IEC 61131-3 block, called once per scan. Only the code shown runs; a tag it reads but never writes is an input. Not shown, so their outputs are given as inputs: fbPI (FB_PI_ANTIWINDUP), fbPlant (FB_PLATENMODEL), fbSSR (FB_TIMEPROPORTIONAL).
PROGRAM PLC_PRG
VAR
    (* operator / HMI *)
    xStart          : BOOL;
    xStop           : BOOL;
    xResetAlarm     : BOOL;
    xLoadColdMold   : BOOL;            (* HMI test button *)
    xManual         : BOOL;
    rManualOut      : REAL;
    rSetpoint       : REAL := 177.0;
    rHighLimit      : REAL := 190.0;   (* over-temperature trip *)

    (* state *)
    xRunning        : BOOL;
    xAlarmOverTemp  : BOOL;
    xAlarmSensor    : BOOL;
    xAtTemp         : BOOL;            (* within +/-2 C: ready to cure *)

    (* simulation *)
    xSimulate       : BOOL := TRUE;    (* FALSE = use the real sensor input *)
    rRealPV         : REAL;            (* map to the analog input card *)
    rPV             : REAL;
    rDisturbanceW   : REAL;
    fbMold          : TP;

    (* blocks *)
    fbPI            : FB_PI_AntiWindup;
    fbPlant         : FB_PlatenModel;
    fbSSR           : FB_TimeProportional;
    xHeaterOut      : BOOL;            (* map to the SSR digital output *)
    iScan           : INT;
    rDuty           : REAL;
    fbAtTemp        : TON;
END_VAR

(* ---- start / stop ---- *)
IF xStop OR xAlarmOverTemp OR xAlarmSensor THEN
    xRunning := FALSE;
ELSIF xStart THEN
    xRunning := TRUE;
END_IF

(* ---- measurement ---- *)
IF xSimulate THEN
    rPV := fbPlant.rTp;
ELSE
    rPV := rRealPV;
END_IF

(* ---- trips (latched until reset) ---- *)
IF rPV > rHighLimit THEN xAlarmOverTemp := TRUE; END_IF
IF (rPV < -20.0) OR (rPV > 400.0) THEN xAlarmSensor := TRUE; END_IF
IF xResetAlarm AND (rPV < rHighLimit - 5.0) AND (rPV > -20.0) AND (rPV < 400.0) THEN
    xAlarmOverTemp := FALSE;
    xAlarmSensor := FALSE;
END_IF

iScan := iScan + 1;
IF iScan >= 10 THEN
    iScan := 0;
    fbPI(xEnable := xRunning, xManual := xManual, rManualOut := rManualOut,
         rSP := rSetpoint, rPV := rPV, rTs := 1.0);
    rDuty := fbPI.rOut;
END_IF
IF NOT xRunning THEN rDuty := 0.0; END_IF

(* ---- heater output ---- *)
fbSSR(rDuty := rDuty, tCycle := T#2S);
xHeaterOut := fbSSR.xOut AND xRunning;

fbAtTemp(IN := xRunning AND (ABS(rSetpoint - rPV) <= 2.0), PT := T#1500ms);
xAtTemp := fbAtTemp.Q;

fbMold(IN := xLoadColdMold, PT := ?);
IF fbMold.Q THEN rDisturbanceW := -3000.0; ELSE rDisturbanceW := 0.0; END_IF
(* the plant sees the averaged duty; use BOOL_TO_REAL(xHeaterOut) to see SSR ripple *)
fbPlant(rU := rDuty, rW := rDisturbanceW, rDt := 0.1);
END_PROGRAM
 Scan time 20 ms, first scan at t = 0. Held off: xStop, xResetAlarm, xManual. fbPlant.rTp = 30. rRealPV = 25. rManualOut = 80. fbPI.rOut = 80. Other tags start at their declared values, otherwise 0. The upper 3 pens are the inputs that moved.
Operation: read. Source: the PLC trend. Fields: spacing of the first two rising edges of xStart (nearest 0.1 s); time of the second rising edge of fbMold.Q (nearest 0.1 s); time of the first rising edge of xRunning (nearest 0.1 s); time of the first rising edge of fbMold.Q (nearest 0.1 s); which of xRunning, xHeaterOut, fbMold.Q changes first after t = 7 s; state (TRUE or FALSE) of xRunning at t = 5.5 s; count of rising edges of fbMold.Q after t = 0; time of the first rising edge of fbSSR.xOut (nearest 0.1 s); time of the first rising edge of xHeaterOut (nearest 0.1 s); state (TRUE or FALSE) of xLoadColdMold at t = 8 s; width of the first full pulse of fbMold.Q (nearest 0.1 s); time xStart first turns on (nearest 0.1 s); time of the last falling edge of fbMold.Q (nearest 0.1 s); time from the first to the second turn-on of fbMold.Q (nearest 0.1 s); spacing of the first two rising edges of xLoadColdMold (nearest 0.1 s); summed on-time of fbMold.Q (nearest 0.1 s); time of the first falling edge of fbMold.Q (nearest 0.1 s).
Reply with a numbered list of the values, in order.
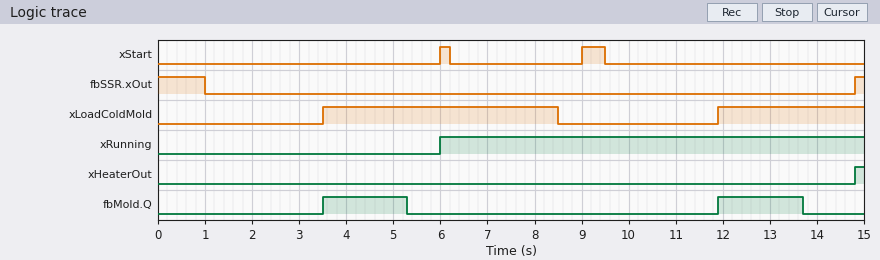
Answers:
1. 3.0 s
2. 11.9 s
3. 6.0 s
4. 3.5 s
5. fbMold.Q
6. FALSE
7. 2
8. 14.8 s
9. 14.8 s
10. TRUE
11. 1.8 s
12. 6.0 s
13. 13.7 s
14. 8.4 s
15. 8.4 s
16. 3.6 s
17. 5.3 s
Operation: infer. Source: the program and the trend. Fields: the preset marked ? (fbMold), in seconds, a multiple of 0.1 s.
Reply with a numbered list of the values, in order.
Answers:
1. 1.8 s
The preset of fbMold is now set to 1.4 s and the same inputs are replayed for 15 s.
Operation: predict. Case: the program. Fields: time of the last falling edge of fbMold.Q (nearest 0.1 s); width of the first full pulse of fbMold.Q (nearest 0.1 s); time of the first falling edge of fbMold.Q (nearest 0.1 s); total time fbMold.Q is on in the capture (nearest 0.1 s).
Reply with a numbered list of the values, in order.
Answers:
1. 13.3 s
2. 1.4 s
3. 4.9 s
4. 2.8 s
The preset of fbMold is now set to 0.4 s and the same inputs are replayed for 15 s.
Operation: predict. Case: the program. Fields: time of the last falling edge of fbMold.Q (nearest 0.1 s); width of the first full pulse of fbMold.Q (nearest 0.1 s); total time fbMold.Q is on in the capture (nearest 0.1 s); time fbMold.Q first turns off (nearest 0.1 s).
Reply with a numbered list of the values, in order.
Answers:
1. 12.3 s
2. 0.4 s
3. 0.8 s
4. 3.9 s
